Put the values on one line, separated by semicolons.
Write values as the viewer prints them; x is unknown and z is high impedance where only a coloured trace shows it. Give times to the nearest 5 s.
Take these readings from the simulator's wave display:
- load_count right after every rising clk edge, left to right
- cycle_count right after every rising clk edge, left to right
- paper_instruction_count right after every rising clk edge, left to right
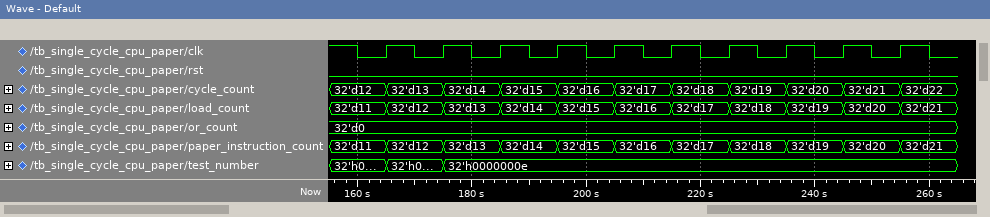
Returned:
32'd12, 32'd13, 32'd14, 32'd15, 32'd16, 32'd17, 32'd18, 32'd19, 32'd20, 32'd21; 32'd13, 32'd14, 32'd15, 32'd16, 32'd17, 32'd18, 32'd19, 32'd20, 32'd21, 32'd22; 32'd12, 32'd13, 32'd14, 32'd15, 32'd16, 32'd17, 32'd18, 32'd19, 32'd20, 32'd21
